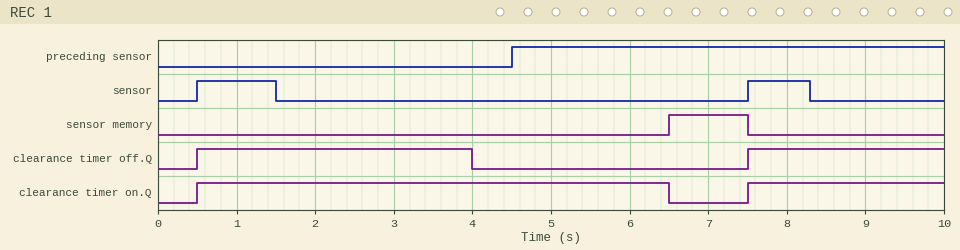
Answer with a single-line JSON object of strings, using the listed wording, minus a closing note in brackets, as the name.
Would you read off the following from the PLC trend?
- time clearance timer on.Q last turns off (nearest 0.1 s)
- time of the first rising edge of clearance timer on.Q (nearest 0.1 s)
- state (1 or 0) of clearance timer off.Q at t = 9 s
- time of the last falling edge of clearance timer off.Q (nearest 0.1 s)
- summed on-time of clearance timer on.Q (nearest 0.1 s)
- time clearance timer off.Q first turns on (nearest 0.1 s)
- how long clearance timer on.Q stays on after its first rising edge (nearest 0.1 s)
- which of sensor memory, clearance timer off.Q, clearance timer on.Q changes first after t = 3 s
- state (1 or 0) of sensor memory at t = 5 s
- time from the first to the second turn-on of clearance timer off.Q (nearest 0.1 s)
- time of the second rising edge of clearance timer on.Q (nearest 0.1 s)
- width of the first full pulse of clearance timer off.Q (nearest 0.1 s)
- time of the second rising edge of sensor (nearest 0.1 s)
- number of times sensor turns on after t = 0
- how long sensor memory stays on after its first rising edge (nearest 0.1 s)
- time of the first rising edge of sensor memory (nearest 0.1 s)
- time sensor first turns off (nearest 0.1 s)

{"time clearance timer on.Q last turns off": "6.5 s", "time of the first rising edge of clearance timer on.Q": "0.5 s", "state (1 or 0) of clearance timer off.Q at t = 9 s": "1", "time of the last falling edge of clearance timer off.Q": "4.0 s", "summed on-time of clearance timer on.Q": "8.5 s", "time clearance timer off.Q first turns on": "0.5 s", "how long clearance timer on.Q stays on after its first rising edge": "6.0 s", "which of sensor memory, clearance timer off.Q, clearance timer on.Q changes first after t = 3 s": "clearance timer off.Q", "state (1 or 0) of sensor memory at t = 5 s": "0", "time from the first to the second turn-on of clearance timer off.Q": "7.0 s", "time of the second rising edge of clearance timer on.Q": "7.5 s", "width of the first full pulse of clearance timer off.Q": "3.5 s", "time of the second rising edge of sensor": "7.5 s", "number of times sensor turns on after t = 0": "2", "how long sensor memory stays on after its first rising edge": "1.0 s", "time of the first rising edge of sensor memory": "6.5 s", "time sensor first turns off": "1.5 s"}
